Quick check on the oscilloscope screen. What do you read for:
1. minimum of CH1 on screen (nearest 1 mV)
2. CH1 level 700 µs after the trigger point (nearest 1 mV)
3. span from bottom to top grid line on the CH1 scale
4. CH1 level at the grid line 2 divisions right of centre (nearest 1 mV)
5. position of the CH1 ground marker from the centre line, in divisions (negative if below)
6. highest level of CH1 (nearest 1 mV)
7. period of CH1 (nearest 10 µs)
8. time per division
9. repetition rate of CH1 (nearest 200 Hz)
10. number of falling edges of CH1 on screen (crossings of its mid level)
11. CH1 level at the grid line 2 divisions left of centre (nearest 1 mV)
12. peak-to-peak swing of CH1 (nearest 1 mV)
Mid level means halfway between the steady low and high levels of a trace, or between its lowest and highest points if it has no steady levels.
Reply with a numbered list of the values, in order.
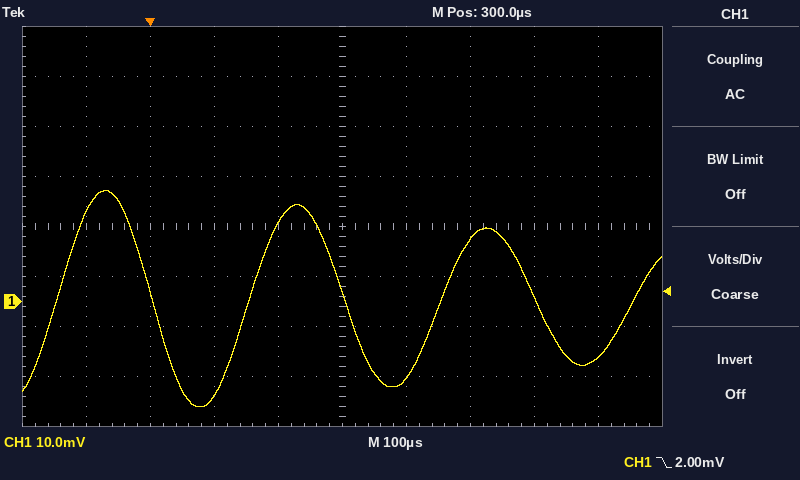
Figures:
1. -21 mV
2. -11 mV
3. 80 mV
4. 12 mV
5. -1.5 div
6. 22 mV
7. 300 µs
8. 100 µs
9. 3.4 kHz
10. 3
11. -19 mV
12. 43 mV
